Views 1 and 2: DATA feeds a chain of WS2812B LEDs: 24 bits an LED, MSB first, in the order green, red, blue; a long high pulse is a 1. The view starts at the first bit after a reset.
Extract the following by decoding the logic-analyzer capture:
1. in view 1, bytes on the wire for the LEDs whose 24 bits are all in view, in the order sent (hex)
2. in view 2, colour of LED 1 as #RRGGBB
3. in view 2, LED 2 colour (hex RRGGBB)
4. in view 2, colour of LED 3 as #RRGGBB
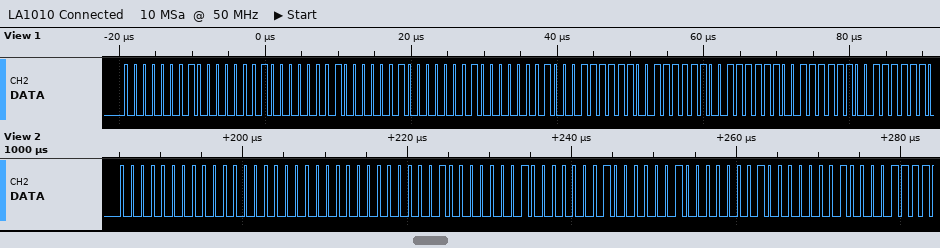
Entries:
01 01 01 02 02 02 3F 3F 3F
#000000
#010101
#020202
